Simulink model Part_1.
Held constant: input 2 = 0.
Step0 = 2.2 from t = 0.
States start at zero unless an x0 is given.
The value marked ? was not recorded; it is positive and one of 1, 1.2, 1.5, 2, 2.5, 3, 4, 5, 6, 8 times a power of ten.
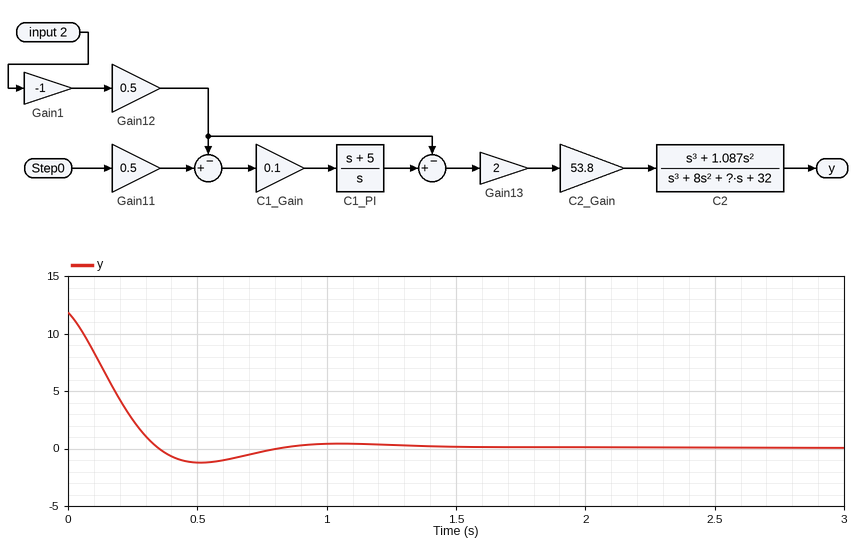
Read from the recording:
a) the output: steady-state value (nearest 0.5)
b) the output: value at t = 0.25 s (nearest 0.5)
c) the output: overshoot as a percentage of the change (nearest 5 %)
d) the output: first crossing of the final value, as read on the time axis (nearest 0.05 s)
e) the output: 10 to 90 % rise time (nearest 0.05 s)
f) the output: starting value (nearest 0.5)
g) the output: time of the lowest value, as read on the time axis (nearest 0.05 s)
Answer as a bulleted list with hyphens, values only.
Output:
- 0.0
- 2.5
- 10 %
- 0.35 s
- 0.25 s
- 12.0
- 0.50 s
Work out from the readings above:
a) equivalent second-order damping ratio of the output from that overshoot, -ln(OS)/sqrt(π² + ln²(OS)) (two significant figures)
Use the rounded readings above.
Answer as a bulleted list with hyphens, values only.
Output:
- 0.59
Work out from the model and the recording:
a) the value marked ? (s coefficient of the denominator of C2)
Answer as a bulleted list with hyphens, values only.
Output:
- 50
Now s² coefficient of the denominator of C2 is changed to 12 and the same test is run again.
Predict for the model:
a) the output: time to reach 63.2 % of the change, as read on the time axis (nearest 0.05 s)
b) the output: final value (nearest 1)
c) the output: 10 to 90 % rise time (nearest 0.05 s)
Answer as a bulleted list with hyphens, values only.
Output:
- 0.15 s
- 0
- 0.30 s
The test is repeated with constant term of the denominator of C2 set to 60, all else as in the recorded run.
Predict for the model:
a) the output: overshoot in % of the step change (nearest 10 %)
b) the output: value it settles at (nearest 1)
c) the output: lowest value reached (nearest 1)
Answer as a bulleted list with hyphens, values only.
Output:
- 20 %
- 0
- -2
